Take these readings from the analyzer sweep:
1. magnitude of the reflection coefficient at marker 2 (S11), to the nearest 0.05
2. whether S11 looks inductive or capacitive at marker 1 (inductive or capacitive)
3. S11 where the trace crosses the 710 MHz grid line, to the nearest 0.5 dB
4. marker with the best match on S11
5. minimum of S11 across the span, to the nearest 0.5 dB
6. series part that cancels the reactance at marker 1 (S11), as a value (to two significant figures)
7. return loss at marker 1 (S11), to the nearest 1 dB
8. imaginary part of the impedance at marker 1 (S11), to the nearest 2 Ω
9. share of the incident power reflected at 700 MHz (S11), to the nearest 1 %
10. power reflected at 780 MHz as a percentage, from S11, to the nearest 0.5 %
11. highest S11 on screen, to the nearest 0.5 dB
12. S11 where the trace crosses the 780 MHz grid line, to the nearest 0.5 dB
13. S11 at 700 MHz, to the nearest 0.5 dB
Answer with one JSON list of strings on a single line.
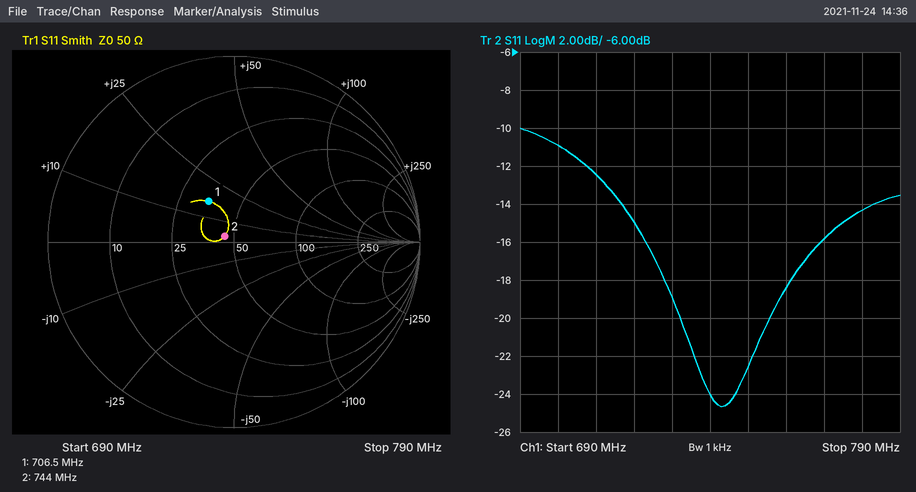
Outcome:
["0.05", "inductive", "-12.5 dB", "marker 2", "-24.5 dB", "14 pF", "12 dB", "+16 Ω", "8 %", "3.5 %", "-10.0 dB", "-14.5 dB", "-11.0 dB"]
